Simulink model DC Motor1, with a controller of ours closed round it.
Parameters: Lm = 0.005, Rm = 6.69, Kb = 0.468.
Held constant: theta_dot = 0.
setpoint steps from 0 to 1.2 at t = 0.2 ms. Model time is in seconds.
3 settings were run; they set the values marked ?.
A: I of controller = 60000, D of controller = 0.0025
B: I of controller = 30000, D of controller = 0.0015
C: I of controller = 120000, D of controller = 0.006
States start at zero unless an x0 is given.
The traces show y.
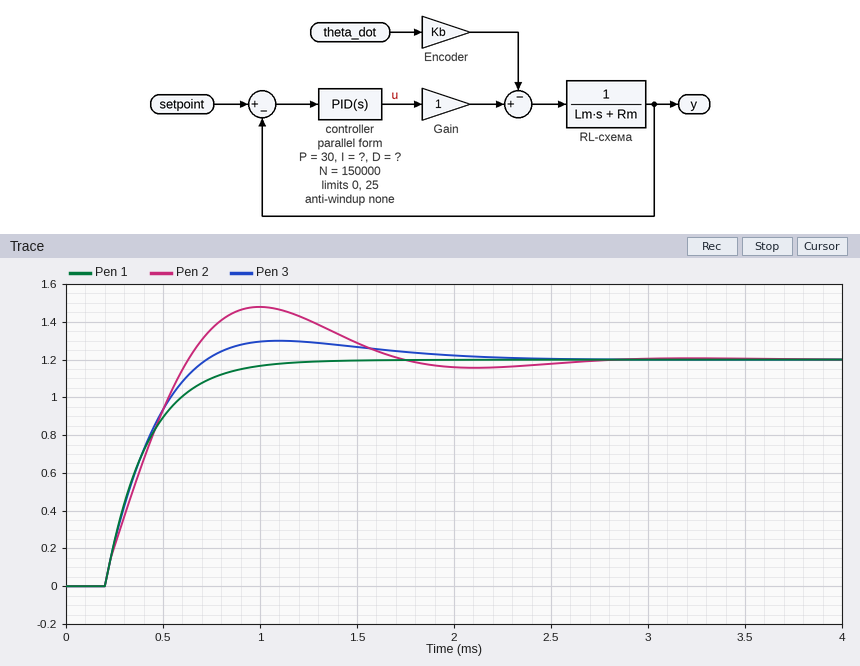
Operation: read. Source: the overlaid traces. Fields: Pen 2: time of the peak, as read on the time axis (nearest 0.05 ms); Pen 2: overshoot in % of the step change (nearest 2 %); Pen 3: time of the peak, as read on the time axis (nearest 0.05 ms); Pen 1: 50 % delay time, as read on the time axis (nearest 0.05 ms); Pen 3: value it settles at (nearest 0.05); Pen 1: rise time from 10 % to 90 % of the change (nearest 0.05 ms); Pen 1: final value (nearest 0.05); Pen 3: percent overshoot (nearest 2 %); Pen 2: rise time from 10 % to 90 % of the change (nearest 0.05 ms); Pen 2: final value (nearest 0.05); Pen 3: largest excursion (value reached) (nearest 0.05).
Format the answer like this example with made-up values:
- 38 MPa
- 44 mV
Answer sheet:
- 1.00 ms
- 24 %
- 1.10 ms
- 0.35 ms
- 1.20
- 0.50 ms
- 1.20
- 8 %
- 0.35 ms
- 1.20
- 1.30
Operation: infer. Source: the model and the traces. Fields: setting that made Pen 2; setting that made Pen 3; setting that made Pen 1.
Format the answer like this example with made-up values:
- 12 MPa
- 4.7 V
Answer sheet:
- C
- A
- B
